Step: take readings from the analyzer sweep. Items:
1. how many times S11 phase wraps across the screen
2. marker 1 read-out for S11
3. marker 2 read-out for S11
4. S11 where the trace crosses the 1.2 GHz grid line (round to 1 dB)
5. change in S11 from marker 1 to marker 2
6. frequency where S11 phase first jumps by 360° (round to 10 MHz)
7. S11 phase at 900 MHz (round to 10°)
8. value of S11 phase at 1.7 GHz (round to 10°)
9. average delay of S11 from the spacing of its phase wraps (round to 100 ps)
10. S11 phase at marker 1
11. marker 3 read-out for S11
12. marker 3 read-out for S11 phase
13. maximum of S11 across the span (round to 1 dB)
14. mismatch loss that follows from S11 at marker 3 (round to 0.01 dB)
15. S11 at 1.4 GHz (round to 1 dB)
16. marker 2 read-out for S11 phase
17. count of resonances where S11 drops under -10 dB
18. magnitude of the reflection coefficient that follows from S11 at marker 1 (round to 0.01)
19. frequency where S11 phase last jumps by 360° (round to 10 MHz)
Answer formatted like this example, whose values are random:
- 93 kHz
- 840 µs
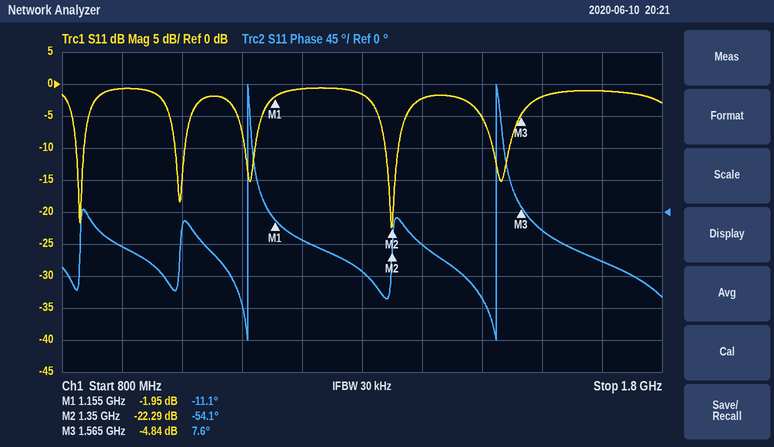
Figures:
- 2
- -1.95 dB
- -22.29 dB
- -1 dB
- -20.34 dB
- 1.11 GHz
- -50°
- -70°
- 2.4 ns
- -11.1°
- -4.84 dB
- 7.6°
- -1 dB
- 1.73 dB
- -2 dB
- -54.1°
- 5
- 0.80
- 1.52 GHz
